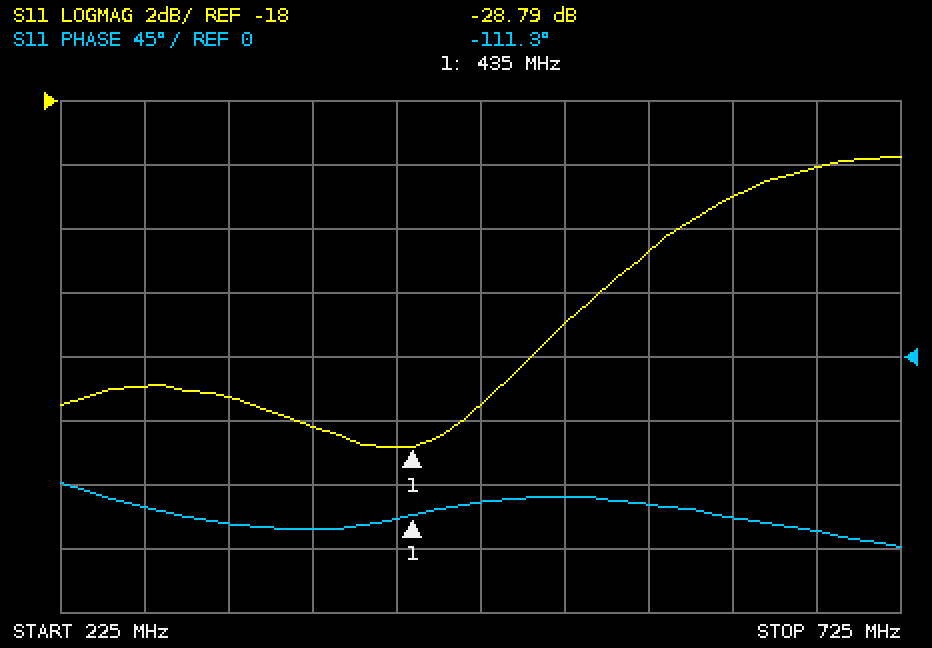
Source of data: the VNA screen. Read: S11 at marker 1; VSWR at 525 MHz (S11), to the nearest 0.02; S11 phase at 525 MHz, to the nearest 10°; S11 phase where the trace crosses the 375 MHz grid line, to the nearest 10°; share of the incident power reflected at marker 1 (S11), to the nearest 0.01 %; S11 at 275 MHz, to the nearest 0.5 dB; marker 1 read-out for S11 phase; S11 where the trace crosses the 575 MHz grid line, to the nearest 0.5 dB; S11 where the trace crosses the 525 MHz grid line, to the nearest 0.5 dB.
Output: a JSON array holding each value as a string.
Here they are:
["-28.79 dB", "1.12", "-100°", "-120°", "0.13 %", "-27.0 dB", "-111.3°", "-22.5 dB", "-25.0 dB"]
